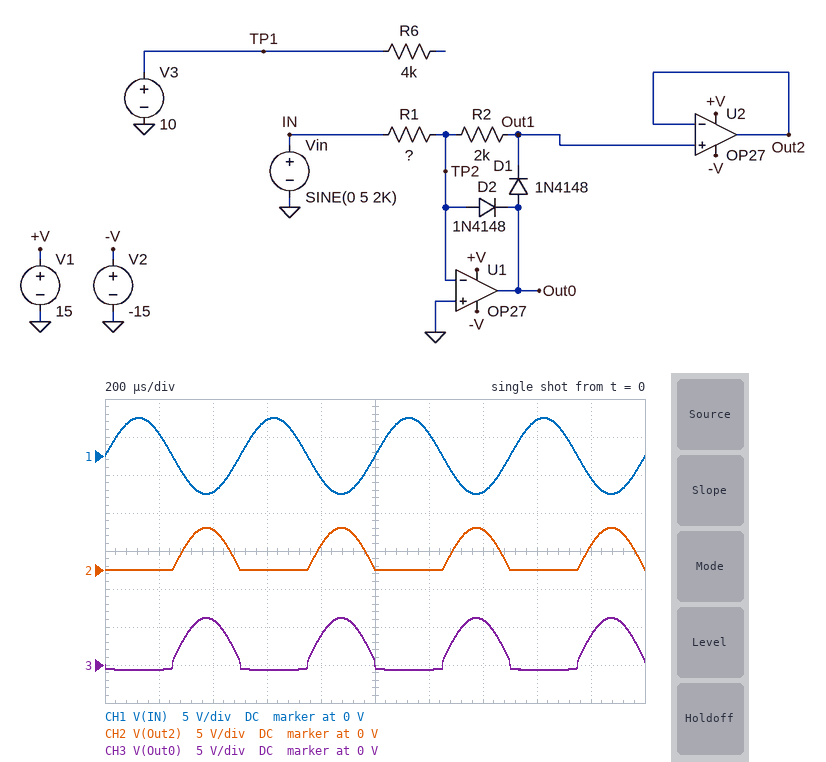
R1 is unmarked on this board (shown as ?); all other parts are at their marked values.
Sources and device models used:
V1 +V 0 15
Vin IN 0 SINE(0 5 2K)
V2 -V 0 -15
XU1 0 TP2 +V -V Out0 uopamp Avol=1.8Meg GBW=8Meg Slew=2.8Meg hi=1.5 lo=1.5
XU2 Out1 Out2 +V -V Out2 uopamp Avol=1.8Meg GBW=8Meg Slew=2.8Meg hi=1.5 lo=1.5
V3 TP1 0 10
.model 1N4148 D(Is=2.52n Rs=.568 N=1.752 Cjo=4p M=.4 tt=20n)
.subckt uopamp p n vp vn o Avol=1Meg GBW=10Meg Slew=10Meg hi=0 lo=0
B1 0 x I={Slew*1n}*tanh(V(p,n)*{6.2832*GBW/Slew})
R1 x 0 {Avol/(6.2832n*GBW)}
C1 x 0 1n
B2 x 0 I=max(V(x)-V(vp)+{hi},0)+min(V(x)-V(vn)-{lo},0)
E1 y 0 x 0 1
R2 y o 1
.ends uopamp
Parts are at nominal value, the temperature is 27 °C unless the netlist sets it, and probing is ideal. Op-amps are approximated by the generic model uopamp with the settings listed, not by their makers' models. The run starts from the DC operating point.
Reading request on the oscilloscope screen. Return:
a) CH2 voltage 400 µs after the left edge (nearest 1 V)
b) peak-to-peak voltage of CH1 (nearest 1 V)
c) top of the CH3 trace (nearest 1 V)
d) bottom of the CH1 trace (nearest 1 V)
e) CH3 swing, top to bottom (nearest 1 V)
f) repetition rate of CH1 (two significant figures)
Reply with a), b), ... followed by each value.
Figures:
a) 5 V
b) 10 V
c) 6 V
d) -5 V
e) 7 V
f) 2.0 kHz
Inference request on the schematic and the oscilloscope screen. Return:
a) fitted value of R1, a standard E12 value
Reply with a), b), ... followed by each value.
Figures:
a) 1.8 kΩ
